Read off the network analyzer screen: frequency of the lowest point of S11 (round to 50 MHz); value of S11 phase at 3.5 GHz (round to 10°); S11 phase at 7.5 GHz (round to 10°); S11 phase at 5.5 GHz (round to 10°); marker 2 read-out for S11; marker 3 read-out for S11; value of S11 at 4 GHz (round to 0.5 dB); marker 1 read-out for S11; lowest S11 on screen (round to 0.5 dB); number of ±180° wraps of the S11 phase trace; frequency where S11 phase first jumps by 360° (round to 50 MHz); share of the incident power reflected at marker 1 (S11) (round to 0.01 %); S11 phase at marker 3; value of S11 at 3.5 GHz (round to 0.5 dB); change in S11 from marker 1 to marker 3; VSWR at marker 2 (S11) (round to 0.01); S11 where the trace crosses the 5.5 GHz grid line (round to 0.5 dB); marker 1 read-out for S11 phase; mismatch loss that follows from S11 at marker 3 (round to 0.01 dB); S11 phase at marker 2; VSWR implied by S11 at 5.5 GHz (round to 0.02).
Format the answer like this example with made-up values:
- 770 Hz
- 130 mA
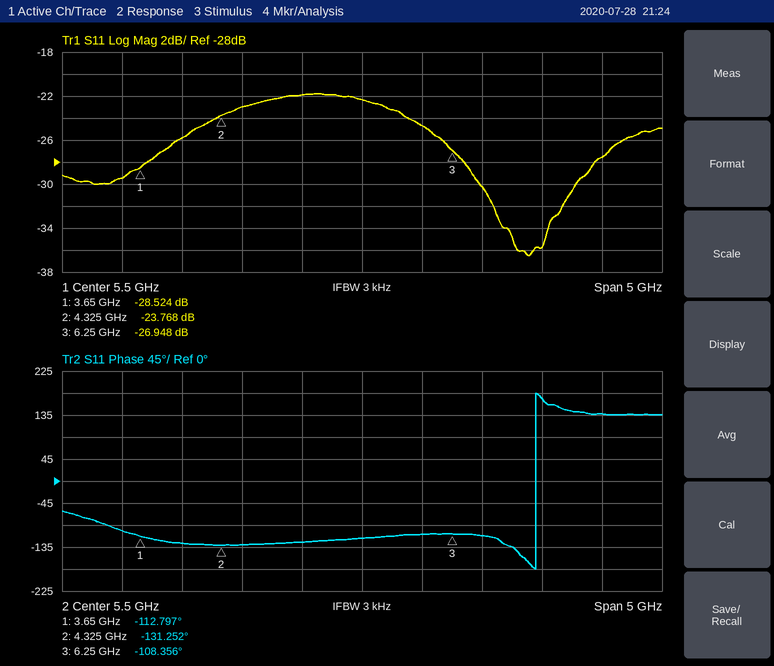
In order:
- 6.90 GHz
- -100°
- 140°
- -120°
- -23.768 dB
- -26.948 dB
- -26.0 dB
- -28.524 dB
- -36.5 dB
- 1
- 6.95 GHz
- 0.14 %
- -108.356°
- -29.5 dB
- 1.576 dB
- 1.14
- -22.5 dB
- -112.797°
- 0.01 dB
- -131.252°
- 1.16
